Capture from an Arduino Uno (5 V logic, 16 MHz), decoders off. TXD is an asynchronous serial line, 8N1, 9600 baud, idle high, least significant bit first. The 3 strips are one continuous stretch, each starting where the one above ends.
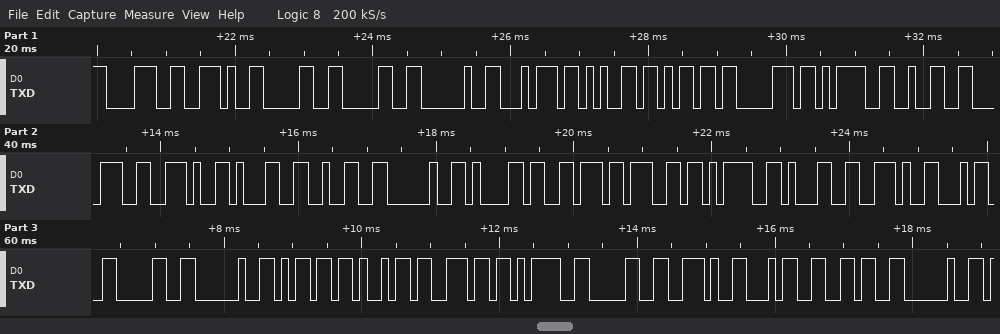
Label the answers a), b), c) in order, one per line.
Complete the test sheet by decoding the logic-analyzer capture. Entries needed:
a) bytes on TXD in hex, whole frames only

a) 38 2E 30 30 20 74 65 6D 70 3D 32 38 2E 31 32 20 61 76 67 3D 31 2E 34 30 20 6D 69 6E 3D 30 2E 34 36 20
